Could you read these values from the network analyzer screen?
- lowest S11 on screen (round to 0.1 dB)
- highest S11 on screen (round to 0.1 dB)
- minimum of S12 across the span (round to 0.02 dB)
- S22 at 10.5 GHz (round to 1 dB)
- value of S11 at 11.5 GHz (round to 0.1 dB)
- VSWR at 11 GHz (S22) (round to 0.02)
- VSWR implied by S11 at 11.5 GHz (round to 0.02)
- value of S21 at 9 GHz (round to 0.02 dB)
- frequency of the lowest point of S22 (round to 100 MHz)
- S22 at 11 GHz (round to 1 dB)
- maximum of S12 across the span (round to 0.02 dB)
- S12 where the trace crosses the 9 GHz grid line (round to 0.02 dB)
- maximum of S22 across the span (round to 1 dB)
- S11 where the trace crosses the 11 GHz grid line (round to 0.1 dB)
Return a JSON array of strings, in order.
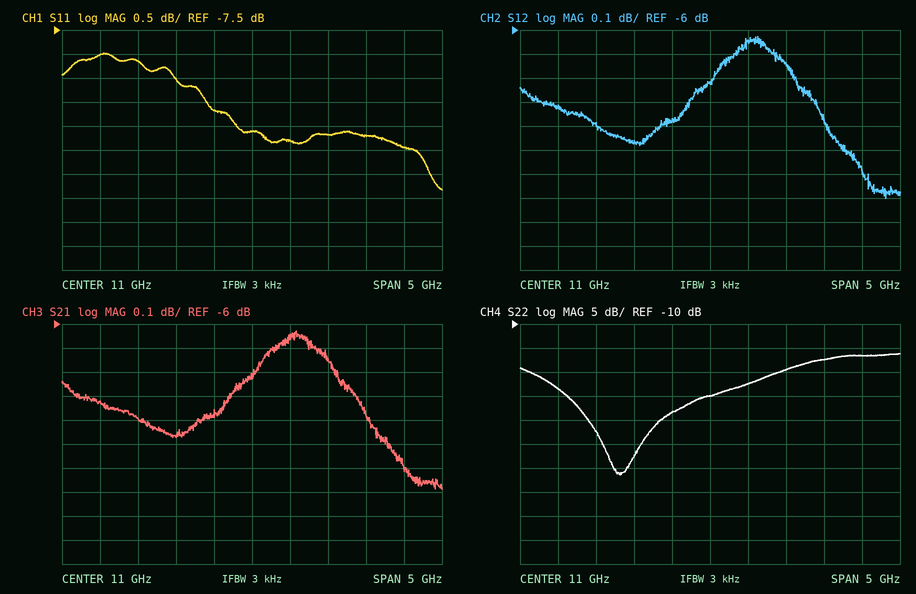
["-10.8 dB", "-8.0 dB", "-6.70 dB", "-28 dB", "-9.8 dB", "1.12", "1.96", "-6.32 dB", "9.8 GHz", "-25 dB", "-6.02 dB", "-6.32 dB", "-16 dB", "-9.6 dB"]
